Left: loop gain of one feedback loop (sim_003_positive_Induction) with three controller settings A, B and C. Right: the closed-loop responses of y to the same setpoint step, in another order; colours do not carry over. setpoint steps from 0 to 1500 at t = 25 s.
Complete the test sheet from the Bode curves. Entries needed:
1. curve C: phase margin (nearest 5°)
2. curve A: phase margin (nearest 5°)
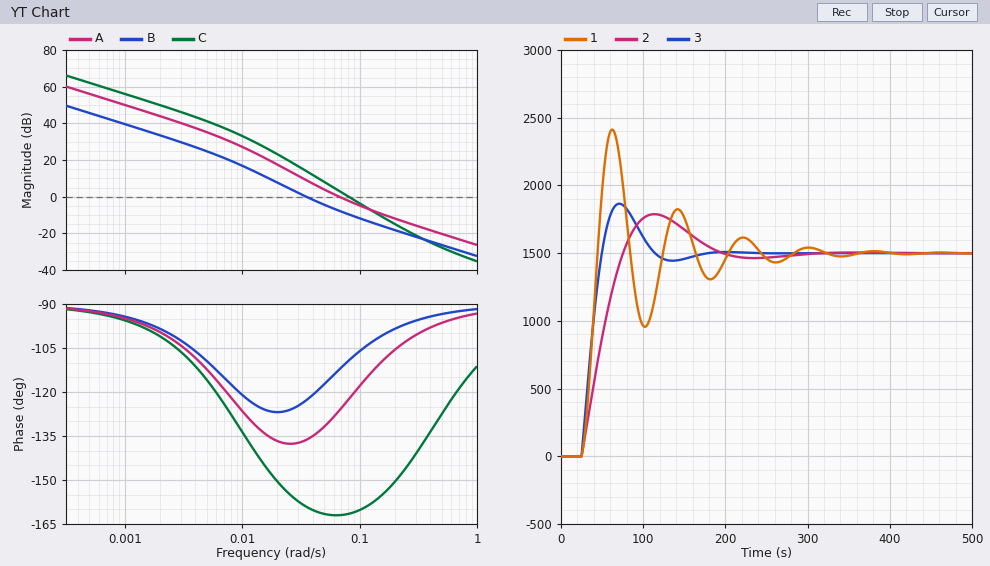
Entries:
20°
55°
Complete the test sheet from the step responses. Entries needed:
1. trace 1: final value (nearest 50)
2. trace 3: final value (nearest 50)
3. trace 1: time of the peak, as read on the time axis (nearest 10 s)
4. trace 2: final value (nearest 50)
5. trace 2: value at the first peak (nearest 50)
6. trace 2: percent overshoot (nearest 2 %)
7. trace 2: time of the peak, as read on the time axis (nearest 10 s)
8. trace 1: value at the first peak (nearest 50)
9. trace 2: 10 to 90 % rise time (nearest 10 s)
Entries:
1500
1500
60 s
1500
1800
20 %
110 s
2400
40 s
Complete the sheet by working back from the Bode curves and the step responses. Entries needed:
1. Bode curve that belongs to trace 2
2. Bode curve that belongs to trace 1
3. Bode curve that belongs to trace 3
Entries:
B
C
A
